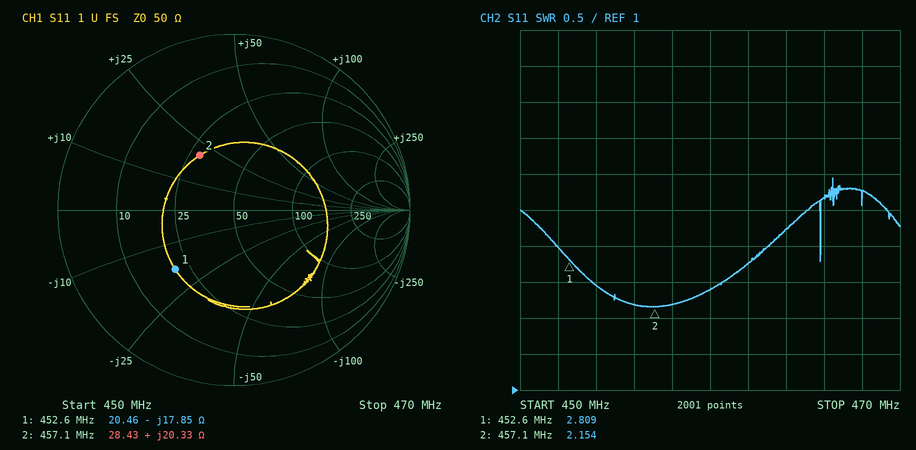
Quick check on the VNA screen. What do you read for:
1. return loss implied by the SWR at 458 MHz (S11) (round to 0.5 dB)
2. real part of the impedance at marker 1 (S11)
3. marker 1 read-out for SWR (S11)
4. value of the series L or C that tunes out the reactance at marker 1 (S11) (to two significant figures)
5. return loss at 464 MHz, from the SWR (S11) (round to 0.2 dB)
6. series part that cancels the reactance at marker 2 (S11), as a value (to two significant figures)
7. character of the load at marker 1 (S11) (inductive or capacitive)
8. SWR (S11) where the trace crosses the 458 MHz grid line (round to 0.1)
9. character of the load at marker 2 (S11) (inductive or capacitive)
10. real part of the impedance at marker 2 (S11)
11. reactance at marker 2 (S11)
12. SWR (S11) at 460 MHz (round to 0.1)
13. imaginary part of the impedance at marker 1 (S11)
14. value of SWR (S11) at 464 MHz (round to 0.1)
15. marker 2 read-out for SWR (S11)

8.5 dB
20.46 Ω
2.809
6.3 nH
5.6 dB
17 pF
capacitive
2.2
inductive
28.43 Ω
+20.33 Ω
2.4
-17.85 Ω
3.2
2.154
